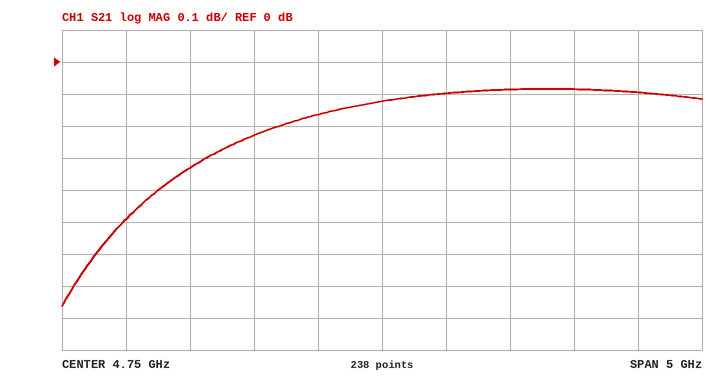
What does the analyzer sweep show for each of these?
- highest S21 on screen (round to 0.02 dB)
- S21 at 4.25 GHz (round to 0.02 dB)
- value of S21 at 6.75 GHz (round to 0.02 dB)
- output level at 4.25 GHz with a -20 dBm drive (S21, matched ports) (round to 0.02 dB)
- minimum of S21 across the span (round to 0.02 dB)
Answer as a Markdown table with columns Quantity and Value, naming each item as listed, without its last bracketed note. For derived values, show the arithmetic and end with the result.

| Quantity | Value |
|---|---|
| highest S21 on screen | -0.08 dB |
| S21 at 4.25 GHz | -0.16 dB |
| value of S21 at 6.75 GHz | -0.10 dB |
| output level at 4.25 GHz with a -20 dBm drive (S21, matched ports) | -20 dBm + (-0.16 dB) = -20.16 dBm |
| minimum of S21 across the span | -0.76 dB |
